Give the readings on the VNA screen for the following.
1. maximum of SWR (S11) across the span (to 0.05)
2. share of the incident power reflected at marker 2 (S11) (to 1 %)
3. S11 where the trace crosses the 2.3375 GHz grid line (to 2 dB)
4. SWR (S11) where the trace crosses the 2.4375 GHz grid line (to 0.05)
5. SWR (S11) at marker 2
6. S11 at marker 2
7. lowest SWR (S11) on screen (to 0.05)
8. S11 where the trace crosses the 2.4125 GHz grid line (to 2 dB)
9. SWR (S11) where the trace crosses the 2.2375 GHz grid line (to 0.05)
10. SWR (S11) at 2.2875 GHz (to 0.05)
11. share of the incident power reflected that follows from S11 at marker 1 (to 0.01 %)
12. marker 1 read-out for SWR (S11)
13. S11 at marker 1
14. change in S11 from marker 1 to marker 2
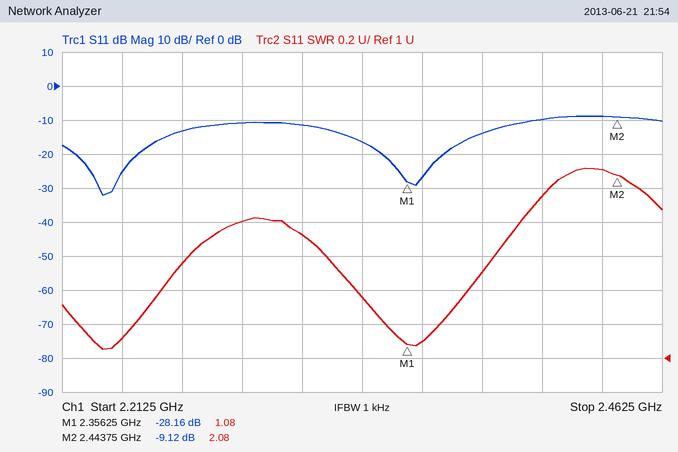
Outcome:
2.10
12 %
-16 dB
2.10
2.08
-9.12 dB
1.05
-10 dB
1.10
1.80
0.15 %
1.08
-28.16 dB
19.04 dB
